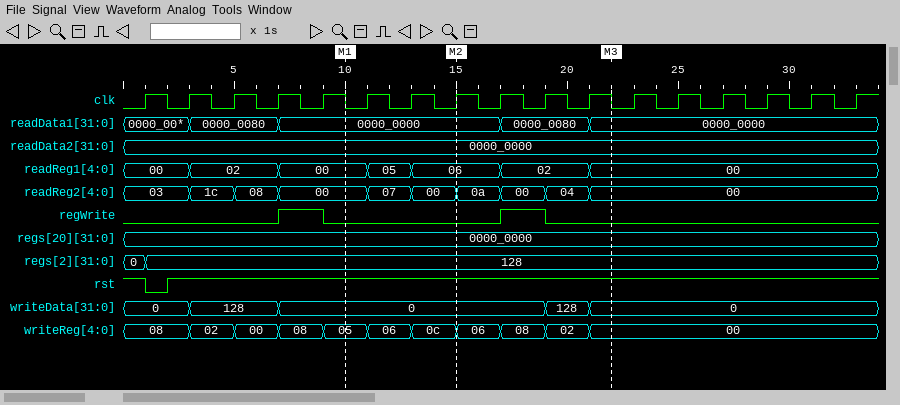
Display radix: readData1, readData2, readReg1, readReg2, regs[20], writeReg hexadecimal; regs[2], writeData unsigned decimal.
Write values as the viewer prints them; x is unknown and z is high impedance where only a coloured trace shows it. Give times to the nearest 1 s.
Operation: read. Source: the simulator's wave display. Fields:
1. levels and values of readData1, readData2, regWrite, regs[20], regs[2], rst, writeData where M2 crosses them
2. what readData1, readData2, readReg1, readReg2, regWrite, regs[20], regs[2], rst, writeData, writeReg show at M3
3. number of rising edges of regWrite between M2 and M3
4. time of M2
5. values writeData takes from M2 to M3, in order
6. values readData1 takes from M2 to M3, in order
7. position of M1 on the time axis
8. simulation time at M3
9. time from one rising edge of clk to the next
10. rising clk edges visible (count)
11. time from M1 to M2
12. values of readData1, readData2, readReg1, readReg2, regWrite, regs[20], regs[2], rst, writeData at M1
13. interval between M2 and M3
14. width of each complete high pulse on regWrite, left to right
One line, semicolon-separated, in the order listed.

readData1=0000_0000, readData2=0000_0000, regWrite=0, regs[20]=0000_0000, regs[2]=128, rst=1, writeData=0; readData1=0000_0000, readData2=0000_0000, readReg1=00, readReg2=00, regWrite=0, regs[20]=0000_0000, regs[2]=128, rst=1, writeData=0, writeReg=00; 1; 15 s; 0, 128, 0; 0000_0000, 0000_0080, 0000_0000; 10 s; 22 s; 2 s; 17; 5 s; readData1=0000_0000, readData2=0000_0000, readReg1=00, readReg2=00, regWrite=0, regs[20]=0000_0000, regs[2]=128, rst=1, writeData=0; 7 s; 2 s, 2 s
